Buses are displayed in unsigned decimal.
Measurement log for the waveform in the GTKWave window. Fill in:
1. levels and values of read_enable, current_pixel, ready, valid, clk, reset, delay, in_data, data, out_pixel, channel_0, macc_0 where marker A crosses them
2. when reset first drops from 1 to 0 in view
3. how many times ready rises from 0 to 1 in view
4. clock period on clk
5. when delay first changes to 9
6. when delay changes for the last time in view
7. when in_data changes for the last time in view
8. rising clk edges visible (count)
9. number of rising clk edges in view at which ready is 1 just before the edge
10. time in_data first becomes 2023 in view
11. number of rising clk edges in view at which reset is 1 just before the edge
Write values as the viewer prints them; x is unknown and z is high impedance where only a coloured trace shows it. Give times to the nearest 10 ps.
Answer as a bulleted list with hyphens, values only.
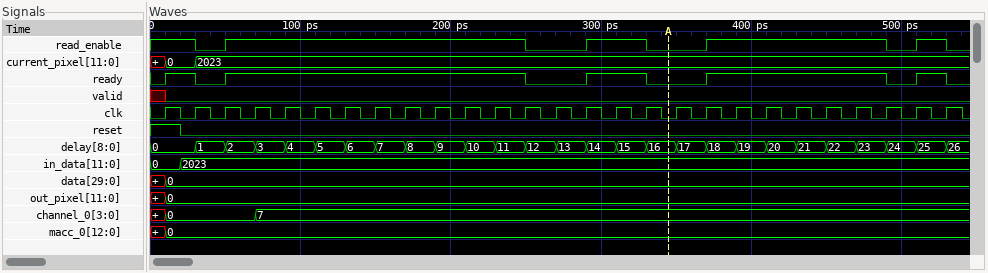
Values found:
- read_enable=0, current_pixel=2023, ready=0, valid=0, clk=0, reset=0, delay=16, in_data=2023, data=0, out_pixel=0, channel_0=7, macc_0=0
- 20 ps
- 5
- 20 ps
- 190 ps
- 530 ps
- 20 ps
- 27
- 20
- 20 ps
- 1
